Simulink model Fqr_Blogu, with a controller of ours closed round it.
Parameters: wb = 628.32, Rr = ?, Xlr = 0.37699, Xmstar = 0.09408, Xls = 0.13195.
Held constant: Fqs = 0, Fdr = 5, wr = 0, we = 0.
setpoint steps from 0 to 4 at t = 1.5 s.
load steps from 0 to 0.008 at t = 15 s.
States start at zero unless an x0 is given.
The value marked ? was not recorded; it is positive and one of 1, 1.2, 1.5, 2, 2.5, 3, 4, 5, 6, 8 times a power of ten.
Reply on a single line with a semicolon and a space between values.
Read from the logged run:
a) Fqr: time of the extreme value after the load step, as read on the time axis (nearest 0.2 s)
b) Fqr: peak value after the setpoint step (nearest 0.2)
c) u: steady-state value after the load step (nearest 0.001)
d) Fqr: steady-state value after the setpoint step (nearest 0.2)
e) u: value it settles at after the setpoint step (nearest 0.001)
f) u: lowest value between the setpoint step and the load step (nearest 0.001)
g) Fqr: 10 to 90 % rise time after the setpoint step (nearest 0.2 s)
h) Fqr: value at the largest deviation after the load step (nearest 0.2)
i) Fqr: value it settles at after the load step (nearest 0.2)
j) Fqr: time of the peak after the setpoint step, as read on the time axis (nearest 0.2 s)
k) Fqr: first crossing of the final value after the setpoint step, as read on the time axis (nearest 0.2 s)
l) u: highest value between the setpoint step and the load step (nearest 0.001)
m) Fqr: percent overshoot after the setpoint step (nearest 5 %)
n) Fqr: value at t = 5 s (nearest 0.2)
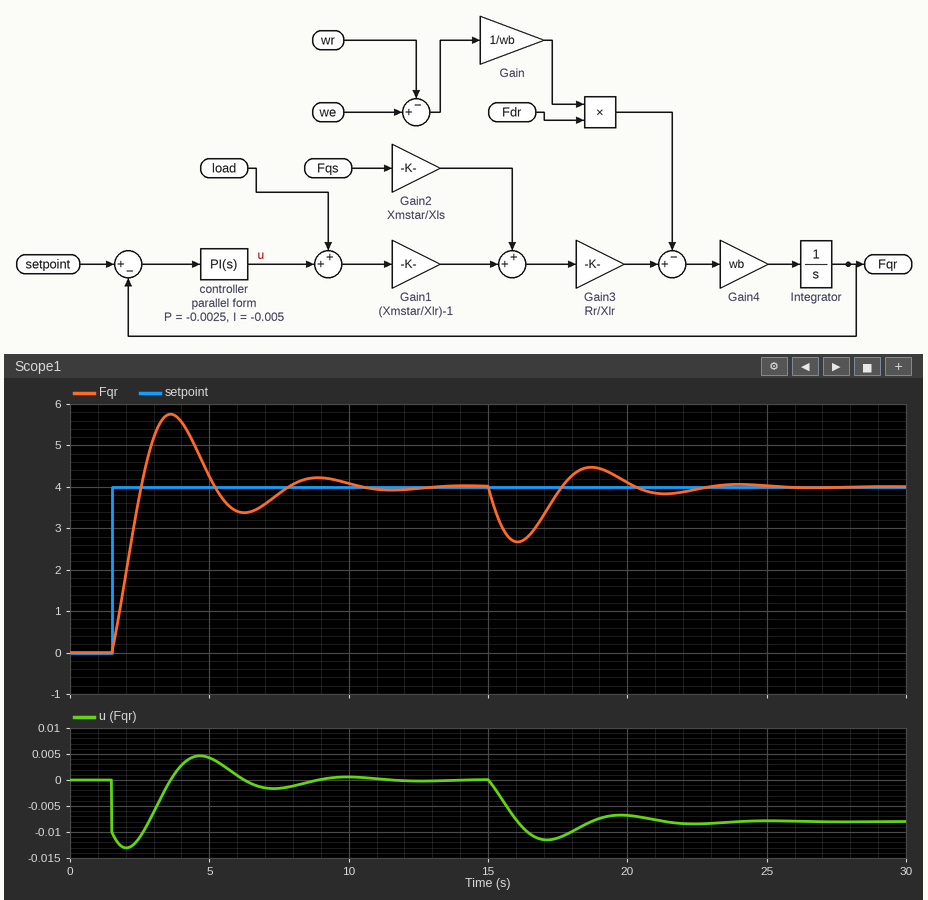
16.0 s; 5.8; -0.008; 4.0; 0.000; -0.013; 0.8 s; 2.6; 4.0; 3.6 s; 2.6 s; 0.005; 45 %; 4.2
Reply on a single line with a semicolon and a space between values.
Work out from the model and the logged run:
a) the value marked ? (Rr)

0.25
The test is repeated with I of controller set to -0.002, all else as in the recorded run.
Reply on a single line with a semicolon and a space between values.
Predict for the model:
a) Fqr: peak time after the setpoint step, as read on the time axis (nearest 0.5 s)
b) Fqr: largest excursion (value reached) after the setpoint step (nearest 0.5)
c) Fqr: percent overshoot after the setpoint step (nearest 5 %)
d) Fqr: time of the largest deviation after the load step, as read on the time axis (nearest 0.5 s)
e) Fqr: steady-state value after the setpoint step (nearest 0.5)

4.5 s; 5.0; 30 %; 16.5 s; 4.0
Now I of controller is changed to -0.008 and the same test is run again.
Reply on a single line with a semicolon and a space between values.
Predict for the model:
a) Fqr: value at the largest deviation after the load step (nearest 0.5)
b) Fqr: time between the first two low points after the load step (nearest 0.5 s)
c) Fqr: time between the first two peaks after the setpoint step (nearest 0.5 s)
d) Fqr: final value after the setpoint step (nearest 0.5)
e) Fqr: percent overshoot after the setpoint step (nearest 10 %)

3.0; 4.0 s; 4.0 s; 4.0; 50 %
